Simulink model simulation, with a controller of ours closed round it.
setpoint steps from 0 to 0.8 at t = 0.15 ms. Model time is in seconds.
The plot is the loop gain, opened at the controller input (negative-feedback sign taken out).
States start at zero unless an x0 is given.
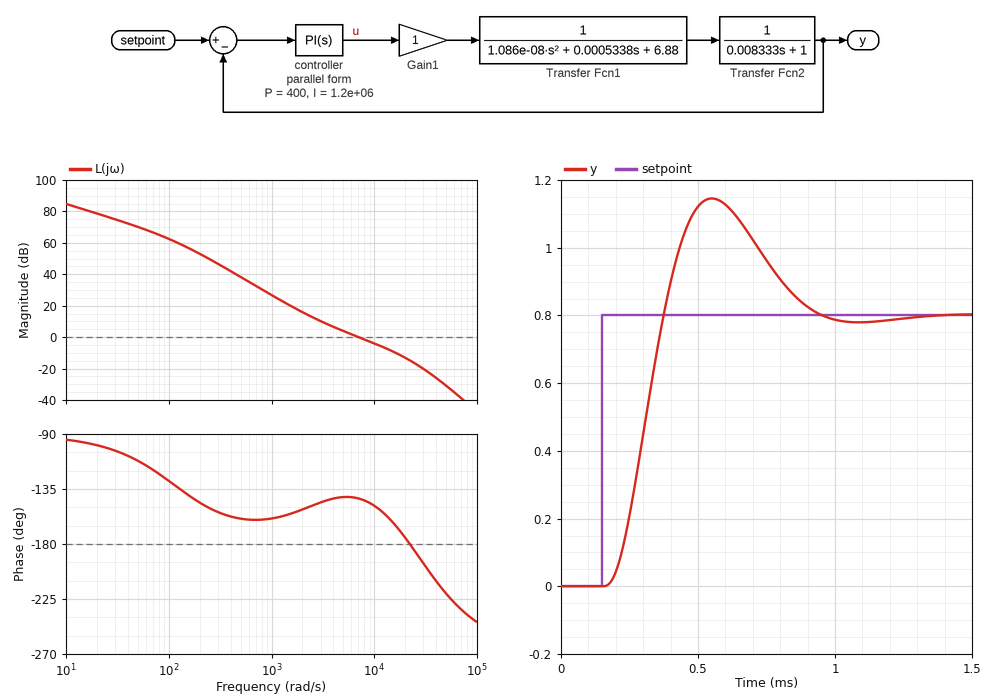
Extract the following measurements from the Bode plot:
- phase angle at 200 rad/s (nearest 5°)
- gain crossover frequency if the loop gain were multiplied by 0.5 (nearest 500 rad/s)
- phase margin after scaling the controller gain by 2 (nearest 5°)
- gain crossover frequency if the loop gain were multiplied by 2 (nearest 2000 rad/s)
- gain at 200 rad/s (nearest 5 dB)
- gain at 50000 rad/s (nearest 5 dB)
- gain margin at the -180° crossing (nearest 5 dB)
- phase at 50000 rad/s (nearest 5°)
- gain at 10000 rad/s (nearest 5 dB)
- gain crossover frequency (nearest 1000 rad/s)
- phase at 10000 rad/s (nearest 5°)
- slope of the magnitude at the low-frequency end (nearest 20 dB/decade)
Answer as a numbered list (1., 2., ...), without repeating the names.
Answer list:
1. -145°
2. 4000 rad/s
3. 25°
4. 12000 rad/s
5. 55 dB
6. -30 dB
7. 15 dB
8. -220°
9. -5 dB
10. 7000 rad/s
11. -150°
12. -20 dB/decade
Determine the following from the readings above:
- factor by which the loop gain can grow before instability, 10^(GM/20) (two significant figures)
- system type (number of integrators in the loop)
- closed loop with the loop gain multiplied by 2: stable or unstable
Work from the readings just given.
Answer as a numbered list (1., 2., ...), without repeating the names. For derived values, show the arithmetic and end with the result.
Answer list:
1. 10^(15 / 20) = 5.6
2. 1
3. stable
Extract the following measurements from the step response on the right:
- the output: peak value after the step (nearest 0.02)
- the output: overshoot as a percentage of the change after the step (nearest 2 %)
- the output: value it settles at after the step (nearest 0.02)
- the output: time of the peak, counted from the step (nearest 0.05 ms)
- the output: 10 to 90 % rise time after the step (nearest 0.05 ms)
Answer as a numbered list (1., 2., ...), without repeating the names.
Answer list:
1. 1.14
2. 44 %
3. 0.80
4. 0.40 ms
5. 0.15 ms
